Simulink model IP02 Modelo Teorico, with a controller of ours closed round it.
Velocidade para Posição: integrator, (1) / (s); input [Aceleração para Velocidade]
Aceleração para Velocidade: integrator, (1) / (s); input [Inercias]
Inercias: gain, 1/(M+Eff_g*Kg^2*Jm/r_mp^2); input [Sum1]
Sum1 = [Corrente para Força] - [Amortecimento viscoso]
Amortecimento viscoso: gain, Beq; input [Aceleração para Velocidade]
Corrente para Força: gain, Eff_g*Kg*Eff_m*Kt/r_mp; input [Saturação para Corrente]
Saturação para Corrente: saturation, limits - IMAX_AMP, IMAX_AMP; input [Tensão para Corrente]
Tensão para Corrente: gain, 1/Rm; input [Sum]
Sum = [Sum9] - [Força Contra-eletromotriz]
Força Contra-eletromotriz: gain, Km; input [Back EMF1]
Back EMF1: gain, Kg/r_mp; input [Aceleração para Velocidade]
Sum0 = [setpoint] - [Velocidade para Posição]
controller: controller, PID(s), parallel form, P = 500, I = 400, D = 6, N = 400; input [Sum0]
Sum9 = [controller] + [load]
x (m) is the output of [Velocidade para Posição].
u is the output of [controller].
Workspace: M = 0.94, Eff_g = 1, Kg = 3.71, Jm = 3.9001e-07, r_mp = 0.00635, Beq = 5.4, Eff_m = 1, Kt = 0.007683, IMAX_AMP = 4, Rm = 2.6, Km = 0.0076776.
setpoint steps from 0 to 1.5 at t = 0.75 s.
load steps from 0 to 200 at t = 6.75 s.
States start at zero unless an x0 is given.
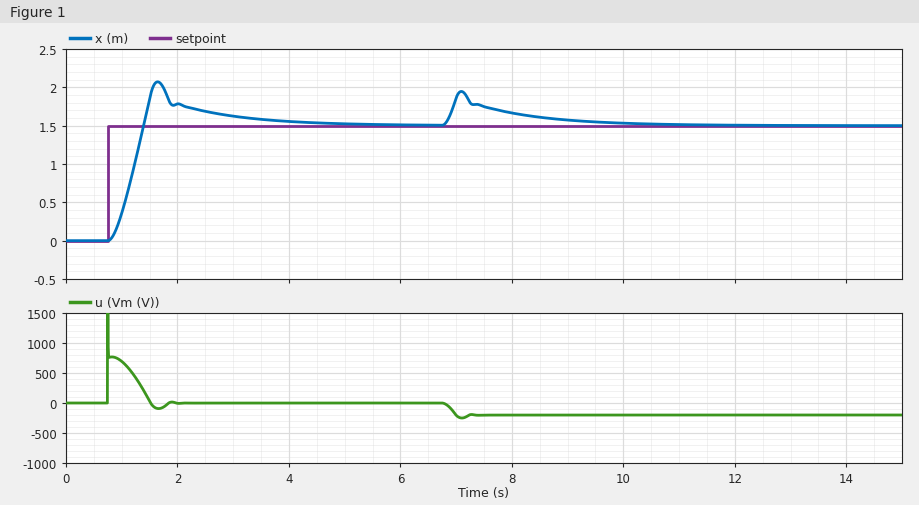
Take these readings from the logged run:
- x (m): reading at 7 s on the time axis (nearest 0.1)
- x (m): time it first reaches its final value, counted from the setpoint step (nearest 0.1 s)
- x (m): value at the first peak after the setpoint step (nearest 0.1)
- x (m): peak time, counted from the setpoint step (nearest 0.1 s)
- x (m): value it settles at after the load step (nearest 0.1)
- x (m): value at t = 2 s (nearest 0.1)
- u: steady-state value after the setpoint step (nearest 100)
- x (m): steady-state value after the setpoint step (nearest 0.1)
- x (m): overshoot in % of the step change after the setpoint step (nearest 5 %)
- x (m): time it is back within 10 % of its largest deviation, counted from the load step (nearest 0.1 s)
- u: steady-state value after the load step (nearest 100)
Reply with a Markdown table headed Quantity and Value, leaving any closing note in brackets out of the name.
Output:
| Quantity | Value |
|---|---|
| x (m): reading at 7 s on the time axis | 1.9 |
| x (m): time it first reaches its final value, counted from the setpoint step | 0.6 s |
| x (m): value at the first peak after the setpoint step | 2.1 |
| x (m): peak time, counted from the setpoint step | 0.9 s |
| x (m): value it settles at after the load step | 1.5 |
| x (m): value at t = 2 s | 1.8 |
| u: steady-state value after the setpoint step | 0 |
| x (m): steady-state value after the setpoint step | 1.5 |
| x (m): overshoot in % of the step change after the setpoint step | 40 % |
| x (m): time it is back within 10 % of its largest deviation, counted from the load step | 2.9 s |
| u: steady-state value after the load step | -200 |
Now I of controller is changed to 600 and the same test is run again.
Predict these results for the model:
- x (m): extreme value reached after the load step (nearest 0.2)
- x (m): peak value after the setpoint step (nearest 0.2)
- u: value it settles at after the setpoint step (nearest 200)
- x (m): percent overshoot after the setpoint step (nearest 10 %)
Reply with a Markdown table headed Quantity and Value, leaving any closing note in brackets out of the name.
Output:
| Quantity | Value |
|---|---|
| x (m): extreme value reached after the load step | 2.0 |
| x (m): peak value after the setpoint step | 2.2 |
| u: value it settles at after the setpoint step | 0 |
| x (m): percent overshoot after the setpoint step | 50 % |
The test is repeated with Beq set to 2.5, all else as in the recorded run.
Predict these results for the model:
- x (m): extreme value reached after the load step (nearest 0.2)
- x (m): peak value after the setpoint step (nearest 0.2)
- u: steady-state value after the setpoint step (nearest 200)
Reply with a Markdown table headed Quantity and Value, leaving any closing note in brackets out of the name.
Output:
| Quantity | Value |
|---|---|
| x (m): extreme value reached after the load step | 2.0 |
| x (m): peak value after the setpoint step | 2.4 |
| u: steady-state value after the setpoint step | 0 |
